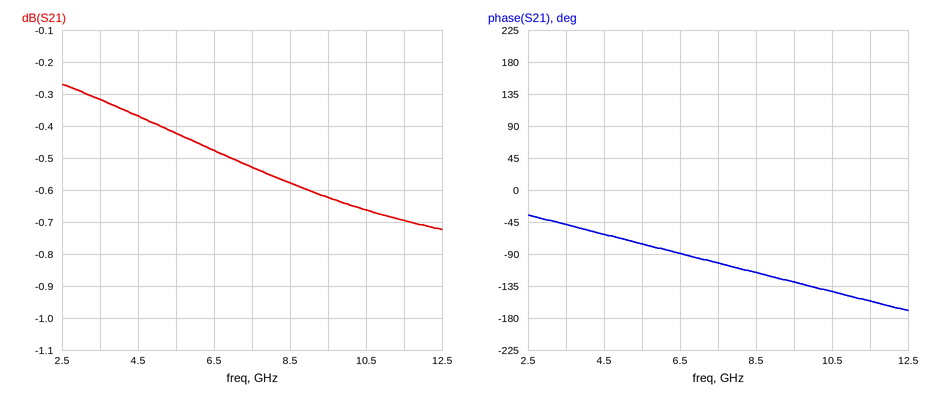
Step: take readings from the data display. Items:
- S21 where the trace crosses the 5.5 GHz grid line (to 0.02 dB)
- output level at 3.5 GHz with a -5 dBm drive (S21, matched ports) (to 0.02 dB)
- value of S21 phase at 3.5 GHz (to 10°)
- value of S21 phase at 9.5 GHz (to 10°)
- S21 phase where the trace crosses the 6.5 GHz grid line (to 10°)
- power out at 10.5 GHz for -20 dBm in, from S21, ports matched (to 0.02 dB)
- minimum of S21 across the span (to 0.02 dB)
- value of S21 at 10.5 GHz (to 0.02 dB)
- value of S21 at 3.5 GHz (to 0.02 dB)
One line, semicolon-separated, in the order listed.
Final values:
-0.42 dB; -5.32 dBm; -50°; -130°; -90°; -20.66 dBm; -0.72 dB; -0.66 dB; -0.32 dB
